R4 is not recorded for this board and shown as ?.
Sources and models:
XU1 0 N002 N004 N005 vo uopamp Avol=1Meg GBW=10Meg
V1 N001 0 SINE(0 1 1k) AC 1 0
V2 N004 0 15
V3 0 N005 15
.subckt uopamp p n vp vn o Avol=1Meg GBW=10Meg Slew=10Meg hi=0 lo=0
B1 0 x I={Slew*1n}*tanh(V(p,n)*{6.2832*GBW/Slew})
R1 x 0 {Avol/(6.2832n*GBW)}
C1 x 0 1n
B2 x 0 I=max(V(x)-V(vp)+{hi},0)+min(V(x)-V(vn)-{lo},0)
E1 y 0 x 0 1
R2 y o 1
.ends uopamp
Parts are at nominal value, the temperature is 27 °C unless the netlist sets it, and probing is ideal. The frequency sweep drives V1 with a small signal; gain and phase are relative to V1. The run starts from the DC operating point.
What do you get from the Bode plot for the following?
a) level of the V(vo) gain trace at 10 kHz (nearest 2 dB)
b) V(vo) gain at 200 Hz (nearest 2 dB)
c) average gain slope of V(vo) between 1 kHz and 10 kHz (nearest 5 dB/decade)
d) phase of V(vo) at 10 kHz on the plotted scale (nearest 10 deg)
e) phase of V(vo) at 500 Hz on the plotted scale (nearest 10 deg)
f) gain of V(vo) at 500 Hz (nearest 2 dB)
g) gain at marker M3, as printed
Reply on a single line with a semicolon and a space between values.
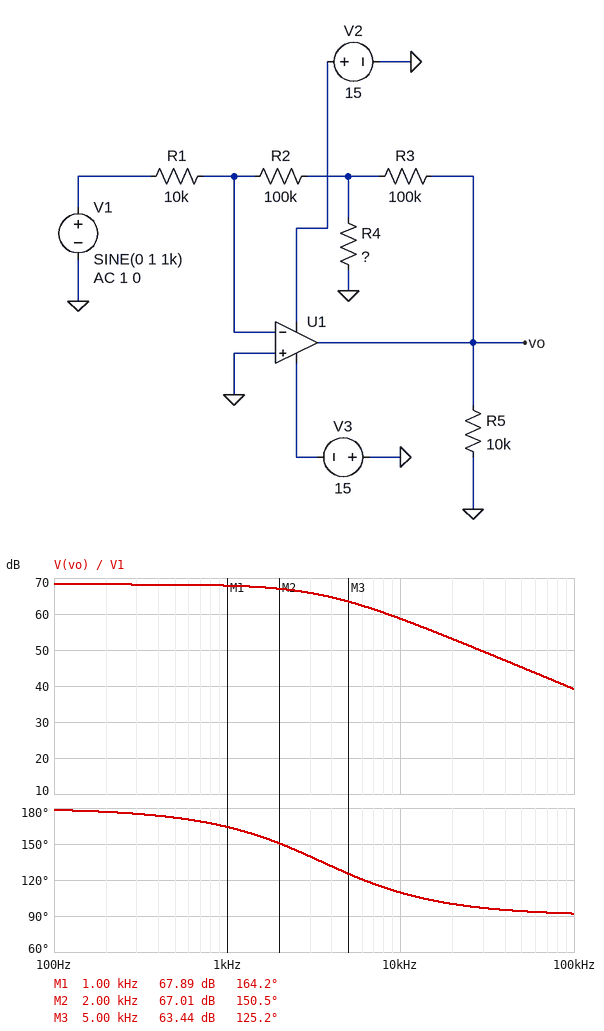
58 dB; 68 dB; -10 dB/decade; 110 deg; 170 deg; 68 dB; 63.44 dB
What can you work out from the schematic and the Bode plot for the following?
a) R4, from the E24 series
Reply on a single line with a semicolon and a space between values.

390 Ω
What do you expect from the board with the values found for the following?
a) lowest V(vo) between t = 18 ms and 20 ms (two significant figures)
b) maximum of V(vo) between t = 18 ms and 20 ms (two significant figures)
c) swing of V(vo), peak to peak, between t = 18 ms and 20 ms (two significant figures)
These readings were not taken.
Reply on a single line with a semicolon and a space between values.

-15 V; 15 V; 30 V
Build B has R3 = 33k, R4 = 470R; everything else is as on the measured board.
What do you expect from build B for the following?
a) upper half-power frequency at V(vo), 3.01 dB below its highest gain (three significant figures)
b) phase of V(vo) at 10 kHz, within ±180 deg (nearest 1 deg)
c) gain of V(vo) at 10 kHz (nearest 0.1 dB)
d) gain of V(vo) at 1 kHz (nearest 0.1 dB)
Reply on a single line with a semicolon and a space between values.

12.7 kHz; 142 deg; 55.0 dB; 57.1 dB
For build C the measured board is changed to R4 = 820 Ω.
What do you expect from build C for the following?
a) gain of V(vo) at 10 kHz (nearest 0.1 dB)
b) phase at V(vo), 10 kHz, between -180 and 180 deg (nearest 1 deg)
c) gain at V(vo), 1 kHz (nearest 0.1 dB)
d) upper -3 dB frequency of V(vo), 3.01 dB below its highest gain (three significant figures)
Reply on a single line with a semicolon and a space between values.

57.3 dB; 126 deg; 61.8 dB; 7.35 kHz
